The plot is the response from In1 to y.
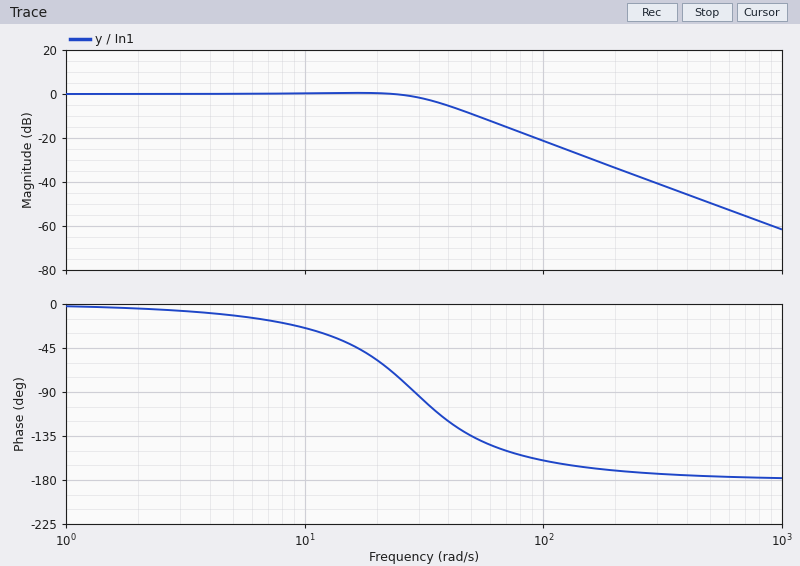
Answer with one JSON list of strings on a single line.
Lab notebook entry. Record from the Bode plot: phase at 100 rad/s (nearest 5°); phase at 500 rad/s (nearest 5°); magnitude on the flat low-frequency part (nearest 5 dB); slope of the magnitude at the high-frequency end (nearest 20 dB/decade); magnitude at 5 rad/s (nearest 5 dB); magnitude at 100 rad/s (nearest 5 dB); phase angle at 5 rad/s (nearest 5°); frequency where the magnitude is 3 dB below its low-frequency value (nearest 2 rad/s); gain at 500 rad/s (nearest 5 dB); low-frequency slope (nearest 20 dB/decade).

["-160°", "-175°", "0 dB", "-40 dB/decade", "0 dB", "-20 dB", "-10°", "34 rad/s", "-50 dB", "0 dB/decade"]
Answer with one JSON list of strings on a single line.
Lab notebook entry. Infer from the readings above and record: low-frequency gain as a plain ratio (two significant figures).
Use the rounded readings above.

["1.0"]
